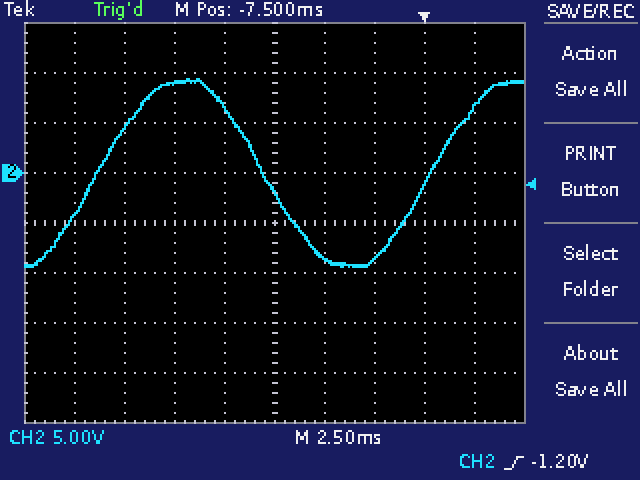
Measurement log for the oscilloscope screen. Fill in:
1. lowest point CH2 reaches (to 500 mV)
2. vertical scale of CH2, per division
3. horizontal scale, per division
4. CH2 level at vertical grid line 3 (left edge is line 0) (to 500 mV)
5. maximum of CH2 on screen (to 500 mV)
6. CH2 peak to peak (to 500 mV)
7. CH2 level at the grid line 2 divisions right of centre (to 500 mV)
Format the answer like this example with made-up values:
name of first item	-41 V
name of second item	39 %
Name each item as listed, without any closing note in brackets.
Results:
lowest point CH2 reaches	-9.5 V
vertical scale of CH2, per division	5 V
horizontal scale, per division	2.5 ms
CH2 level at vertical grid line 3 (left edge is line 0)	9.0 V
maximum of CH2 on screen	9.5 V
CH2 peak to peak	19.0 V
CH2 level at the grid line 2 divisions right of centre	-8.5 V
